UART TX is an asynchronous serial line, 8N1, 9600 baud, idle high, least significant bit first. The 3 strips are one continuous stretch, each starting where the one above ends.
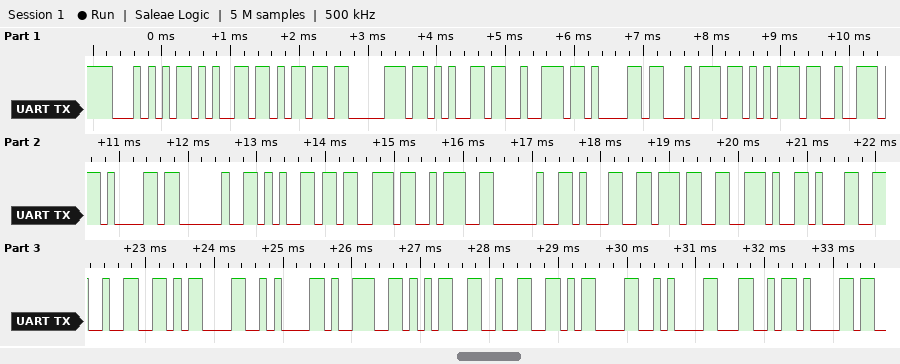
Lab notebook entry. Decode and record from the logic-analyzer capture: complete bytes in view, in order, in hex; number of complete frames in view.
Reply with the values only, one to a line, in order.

54 65 6D 70 65 72 61 74 75 72 61 20 65 73 3A 20 31 37 2E 31 32 0D 0A 39 35 32 0D 0A 4C 61
30
